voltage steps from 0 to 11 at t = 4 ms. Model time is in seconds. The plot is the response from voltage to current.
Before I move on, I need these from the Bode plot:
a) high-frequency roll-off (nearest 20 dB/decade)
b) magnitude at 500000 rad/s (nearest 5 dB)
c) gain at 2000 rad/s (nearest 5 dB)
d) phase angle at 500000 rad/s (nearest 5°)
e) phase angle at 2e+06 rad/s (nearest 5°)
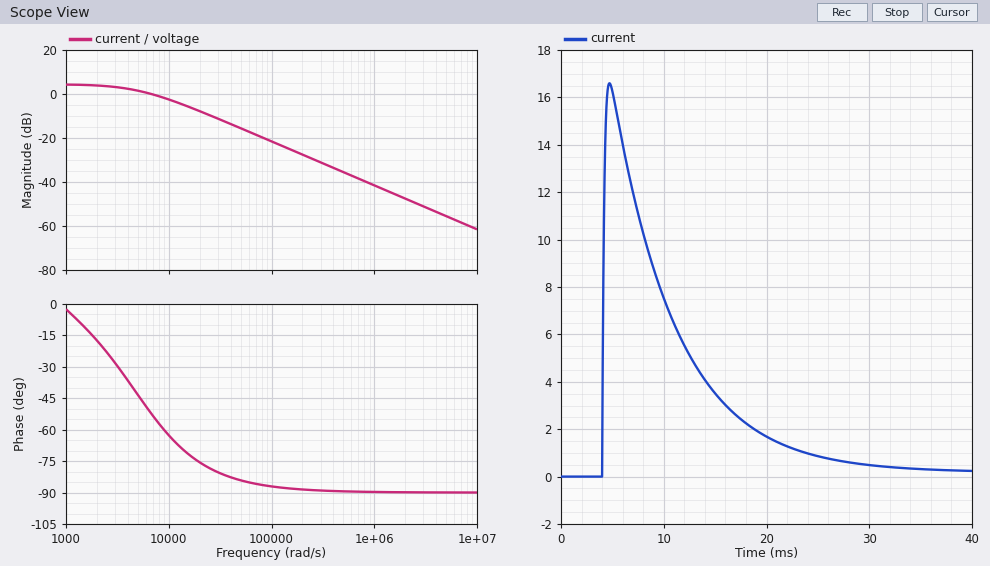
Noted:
-20 dB/decade
-35 dB
5 dB
-90°
-90°
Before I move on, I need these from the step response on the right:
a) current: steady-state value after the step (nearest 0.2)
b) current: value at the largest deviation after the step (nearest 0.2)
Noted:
0.2
16.6
